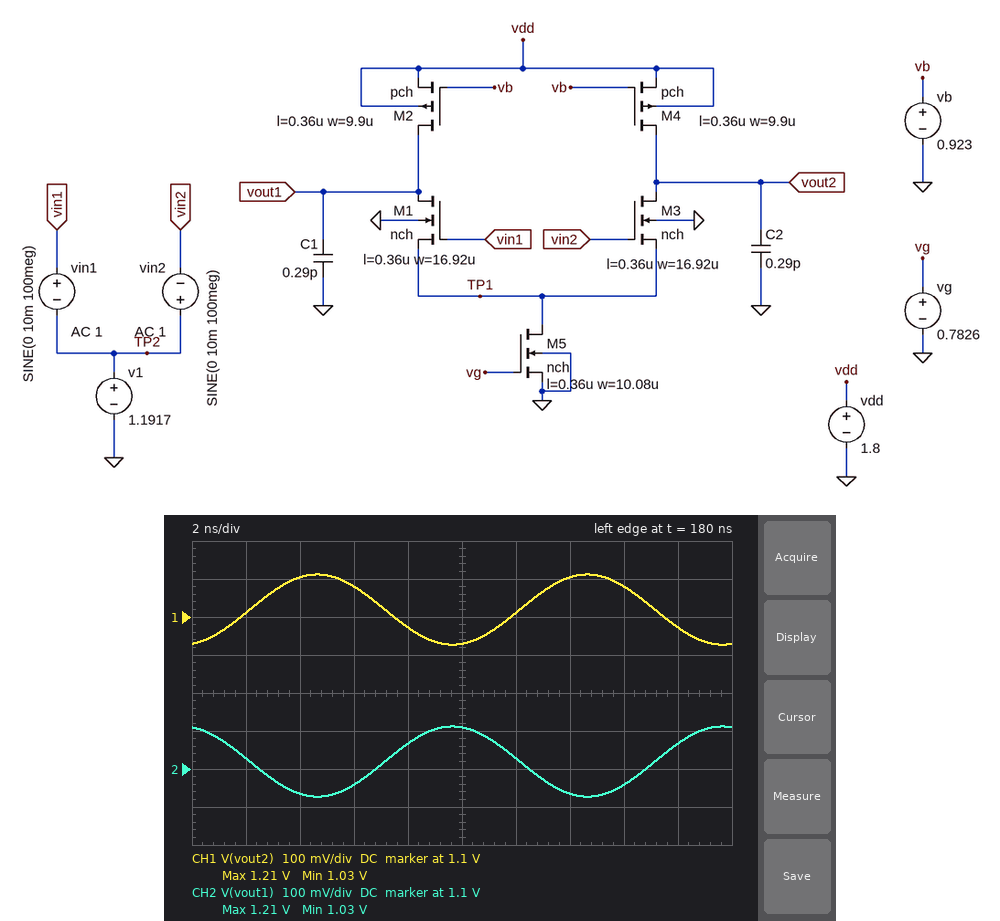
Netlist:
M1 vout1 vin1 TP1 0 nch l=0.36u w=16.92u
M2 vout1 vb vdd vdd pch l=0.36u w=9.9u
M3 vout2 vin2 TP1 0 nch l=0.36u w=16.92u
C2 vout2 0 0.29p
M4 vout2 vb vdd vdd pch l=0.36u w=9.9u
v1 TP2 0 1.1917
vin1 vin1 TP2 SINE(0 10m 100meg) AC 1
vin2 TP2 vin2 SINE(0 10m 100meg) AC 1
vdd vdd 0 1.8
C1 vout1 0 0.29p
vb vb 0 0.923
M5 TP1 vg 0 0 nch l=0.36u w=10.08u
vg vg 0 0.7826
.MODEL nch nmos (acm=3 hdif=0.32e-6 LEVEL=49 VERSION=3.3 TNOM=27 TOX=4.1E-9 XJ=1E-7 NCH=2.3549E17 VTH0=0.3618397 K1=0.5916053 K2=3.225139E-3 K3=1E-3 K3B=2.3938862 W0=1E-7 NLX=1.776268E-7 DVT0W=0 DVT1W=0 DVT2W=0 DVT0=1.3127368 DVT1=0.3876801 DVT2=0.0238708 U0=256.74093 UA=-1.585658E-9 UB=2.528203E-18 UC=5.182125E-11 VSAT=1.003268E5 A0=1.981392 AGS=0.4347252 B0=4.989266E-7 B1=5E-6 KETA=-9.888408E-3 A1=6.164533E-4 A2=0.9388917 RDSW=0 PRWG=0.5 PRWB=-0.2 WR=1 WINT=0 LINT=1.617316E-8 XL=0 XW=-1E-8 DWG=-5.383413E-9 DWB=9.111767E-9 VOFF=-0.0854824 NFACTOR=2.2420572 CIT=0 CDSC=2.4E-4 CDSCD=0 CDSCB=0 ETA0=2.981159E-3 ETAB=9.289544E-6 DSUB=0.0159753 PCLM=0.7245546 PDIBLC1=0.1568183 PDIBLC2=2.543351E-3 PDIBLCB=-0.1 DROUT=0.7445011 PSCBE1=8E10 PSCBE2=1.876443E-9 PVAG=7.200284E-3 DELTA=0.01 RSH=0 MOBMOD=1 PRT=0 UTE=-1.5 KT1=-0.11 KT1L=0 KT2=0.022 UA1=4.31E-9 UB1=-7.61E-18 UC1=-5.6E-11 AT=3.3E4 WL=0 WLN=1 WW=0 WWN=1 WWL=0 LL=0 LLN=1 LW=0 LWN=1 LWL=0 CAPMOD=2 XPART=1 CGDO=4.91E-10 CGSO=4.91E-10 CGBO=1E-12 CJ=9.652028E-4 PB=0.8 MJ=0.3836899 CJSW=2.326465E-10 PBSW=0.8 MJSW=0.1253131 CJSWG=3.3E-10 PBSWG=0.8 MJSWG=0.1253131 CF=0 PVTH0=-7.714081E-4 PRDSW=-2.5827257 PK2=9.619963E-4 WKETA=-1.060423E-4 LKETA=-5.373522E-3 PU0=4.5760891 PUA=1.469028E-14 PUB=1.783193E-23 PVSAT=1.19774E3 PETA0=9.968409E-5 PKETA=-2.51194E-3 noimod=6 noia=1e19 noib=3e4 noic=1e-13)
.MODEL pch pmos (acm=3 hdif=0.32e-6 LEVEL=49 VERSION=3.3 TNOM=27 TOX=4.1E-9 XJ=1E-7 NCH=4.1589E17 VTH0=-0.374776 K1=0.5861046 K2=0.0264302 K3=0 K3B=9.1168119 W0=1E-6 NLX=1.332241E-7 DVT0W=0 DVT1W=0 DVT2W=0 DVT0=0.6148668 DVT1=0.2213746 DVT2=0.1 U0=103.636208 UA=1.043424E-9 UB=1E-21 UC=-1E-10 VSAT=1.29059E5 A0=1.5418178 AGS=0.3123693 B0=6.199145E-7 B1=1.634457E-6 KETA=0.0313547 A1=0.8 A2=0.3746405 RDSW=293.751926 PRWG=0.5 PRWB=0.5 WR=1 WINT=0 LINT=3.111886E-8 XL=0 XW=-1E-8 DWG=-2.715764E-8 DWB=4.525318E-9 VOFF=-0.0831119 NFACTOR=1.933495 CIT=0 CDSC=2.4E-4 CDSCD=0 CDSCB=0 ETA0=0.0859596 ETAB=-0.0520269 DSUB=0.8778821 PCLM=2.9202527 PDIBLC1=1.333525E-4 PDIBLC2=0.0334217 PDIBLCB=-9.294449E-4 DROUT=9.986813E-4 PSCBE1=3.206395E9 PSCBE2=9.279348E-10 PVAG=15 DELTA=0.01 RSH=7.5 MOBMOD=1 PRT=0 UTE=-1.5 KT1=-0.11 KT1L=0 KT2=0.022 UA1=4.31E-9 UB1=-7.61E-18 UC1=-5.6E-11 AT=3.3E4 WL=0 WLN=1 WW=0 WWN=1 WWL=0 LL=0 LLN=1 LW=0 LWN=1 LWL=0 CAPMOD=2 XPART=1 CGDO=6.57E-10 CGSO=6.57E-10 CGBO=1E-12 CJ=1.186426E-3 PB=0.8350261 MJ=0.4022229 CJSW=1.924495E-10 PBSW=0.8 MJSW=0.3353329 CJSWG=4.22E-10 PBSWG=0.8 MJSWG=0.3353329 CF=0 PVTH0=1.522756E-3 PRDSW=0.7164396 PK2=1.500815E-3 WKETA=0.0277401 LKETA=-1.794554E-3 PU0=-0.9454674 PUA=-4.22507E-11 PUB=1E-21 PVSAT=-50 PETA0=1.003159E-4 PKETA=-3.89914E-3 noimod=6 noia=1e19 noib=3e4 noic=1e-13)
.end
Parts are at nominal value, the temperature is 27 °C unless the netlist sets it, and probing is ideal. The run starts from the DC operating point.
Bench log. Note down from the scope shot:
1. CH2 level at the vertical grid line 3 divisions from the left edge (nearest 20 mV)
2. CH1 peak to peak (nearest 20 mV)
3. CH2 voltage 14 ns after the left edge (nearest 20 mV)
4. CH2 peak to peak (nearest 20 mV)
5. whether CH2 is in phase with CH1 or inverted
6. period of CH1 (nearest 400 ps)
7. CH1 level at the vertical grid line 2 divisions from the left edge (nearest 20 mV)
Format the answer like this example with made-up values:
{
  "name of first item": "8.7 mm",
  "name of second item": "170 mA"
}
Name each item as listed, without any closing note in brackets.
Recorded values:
{
  "CH2 level at the vertical grid line 3 divisions from the left edge": "1.06 V",
  "CH1 peak to peak": "180 mV",
  "CH2 voltage 14 ns after the left edge": "1.04 V",
  "CH2 peak to peak": "180 mV",
  "whether CH2 is in phase with CH1 or inverted": "inverted",
  "period of CH1": "10.0 ns",
  "CH1 level at the vertical grid line 2 divisions from the left edge": "1.20 V"
}
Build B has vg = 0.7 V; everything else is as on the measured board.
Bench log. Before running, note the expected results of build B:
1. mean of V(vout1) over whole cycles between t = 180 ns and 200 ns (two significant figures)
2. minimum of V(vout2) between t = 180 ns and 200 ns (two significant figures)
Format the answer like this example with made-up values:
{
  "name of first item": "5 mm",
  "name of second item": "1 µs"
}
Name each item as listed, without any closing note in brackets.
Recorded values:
{
  "mean of V(vout1) over whole cycles between t = 180 ns and 200 ns": "1.7 V",
  "minimum of V(vout2) between t = 180 ns and 200 ns": "1.6 V"
}
